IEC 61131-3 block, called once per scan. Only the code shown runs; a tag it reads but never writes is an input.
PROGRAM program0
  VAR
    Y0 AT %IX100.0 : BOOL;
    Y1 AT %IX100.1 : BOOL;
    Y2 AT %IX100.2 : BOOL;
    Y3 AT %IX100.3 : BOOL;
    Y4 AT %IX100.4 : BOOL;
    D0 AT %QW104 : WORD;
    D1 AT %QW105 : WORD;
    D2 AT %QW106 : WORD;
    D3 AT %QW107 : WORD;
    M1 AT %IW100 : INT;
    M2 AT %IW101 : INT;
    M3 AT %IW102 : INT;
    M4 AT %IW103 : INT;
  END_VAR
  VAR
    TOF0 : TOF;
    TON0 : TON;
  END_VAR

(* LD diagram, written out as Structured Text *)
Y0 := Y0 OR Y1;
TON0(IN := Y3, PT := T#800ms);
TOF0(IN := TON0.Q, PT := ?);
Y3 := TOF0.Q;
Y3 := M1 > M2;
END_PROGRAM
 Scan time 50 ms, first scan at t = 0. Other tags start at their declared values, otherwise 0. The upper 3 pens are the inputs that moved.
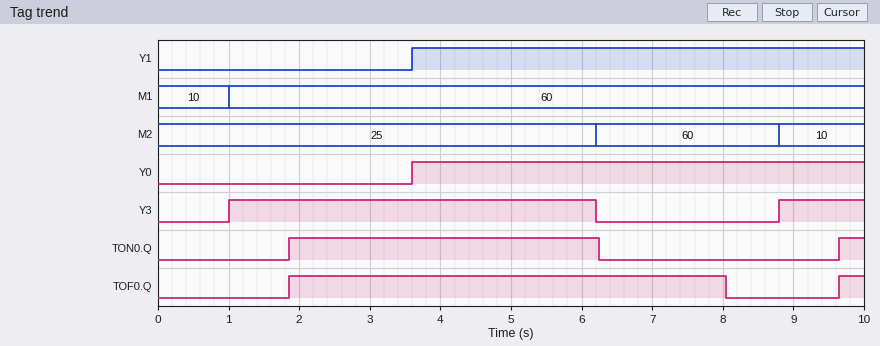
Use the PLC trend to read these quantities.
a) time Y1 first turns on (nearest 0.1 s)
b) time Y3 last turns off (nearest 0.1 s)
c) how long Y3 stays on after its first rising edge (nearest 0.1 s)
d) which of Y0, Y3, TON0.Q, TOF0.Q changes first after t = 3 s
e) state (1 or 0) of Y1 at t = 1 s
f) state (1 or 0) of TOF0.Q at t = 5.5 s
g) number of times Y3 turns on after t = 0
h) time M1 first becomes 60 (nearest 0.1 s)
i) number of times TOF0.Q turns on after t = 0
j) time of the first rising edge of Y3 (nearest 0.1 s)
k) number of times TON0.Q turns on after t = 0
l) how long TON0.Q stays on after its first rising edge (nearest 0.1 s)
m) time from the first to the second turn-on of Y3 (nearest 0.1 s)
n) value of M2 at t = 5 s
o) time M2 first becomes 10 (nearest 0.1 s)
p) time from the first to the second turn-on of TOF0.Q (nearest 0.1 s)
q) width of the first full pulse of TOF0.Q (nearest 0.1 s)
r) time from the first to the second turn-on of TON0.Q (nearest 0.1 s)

3.6 s
6.2 s
5.2 s
Y0
0
1
2
1.0 s
2
1.0 s
2
4.4 s
7.8 s
25
8.8 s
7.8 s
6.2 s
7.8 s
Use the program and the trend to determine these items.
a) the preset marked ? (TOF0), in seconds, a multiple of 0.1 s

1.8 s
